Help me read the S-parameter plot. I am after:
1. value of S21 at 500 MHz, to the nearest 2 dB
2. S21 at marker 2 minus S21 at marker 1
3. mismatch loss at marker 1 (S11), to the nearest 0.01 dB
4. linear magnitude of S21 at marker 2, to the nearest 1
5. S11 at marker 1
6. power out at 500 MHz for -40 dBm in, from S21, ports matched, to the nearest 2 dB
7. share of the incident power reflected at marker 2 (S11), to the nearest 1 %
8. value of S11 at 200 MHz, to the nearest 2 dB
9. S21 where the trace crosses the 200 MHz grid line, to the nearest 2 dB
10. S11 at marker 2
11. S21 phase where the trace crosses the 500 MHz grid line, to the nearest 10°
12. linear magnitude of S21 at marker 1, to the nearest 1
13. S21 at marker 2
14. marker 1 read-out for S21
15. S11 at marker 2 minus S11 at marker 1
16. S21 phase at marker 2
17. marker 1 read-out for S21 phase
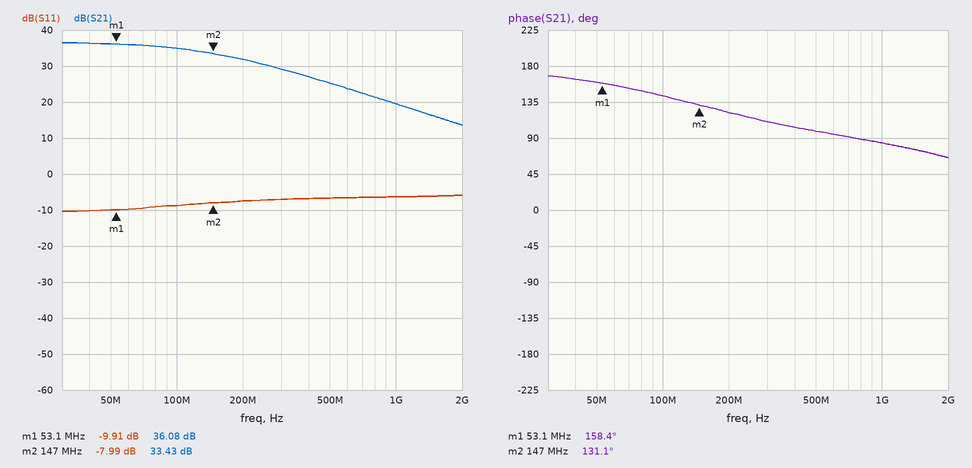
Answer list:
26 dB
-2.65 dB
0.47 dB
47
-9.91 dB
-14 dBm
16 %
-8 dB
32 dB
-7.99 dB
100°
64
33.43 dB
36.08 dB
1.92 dB
131.1°
158.4°
